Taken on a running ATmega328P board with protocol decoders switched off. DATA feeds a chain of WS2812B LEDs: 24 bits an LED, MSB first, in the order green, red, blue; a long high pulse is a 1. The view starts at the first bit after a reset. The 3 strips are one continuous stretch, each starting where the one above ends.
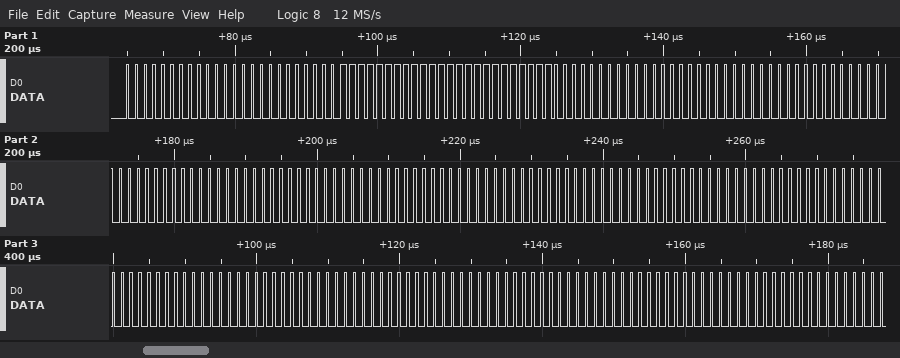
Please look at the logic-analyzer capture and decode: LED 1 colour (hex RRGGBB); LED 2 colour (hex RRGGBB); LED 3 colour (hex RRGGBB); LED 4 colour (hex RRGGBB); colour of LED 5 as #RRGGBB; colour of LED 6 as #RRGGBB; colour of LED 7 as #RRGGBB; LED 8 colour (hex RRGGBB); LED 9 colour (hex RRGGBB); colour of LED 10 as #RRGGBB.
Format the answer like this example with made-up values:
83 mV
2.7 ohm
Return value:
#000000
#FFFFFF
#000000
#000000
#000000
#000000
#000000
#000000
#000000
#000000
